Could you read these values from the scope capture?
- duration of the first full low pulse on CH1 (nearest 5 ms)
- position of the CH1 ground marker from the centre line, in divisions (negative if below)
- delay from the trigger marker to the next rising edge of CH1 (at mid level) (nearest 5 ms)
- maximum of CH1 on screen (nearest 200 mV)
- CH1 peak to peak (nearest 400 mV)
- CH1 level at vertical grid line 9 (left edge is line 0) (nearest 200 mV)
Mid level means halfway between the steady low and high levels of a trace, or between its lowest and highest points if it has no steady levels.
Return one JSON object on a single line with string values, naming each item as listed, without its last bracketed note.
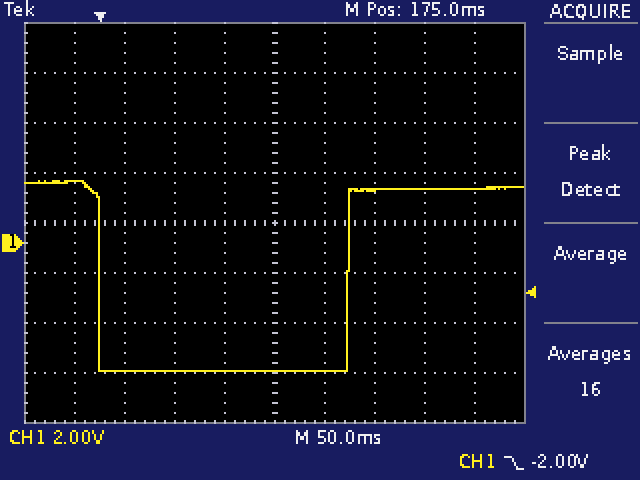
{"duration of the first full low pulse on CH1": "250 ms", "position of the CH1 ground marker from the centre line, in divisions": "-0.4 div", "delay from the trigger marker to the next rising edge of CH1 (at mid level)": "250 ms", "maximum of CH1 on screen": "2.4 V", "CH1 peak to peak": "7.6 V", "CH1 level at vertical grid line 9 (left edge is line 0)": "2.2 V"}
